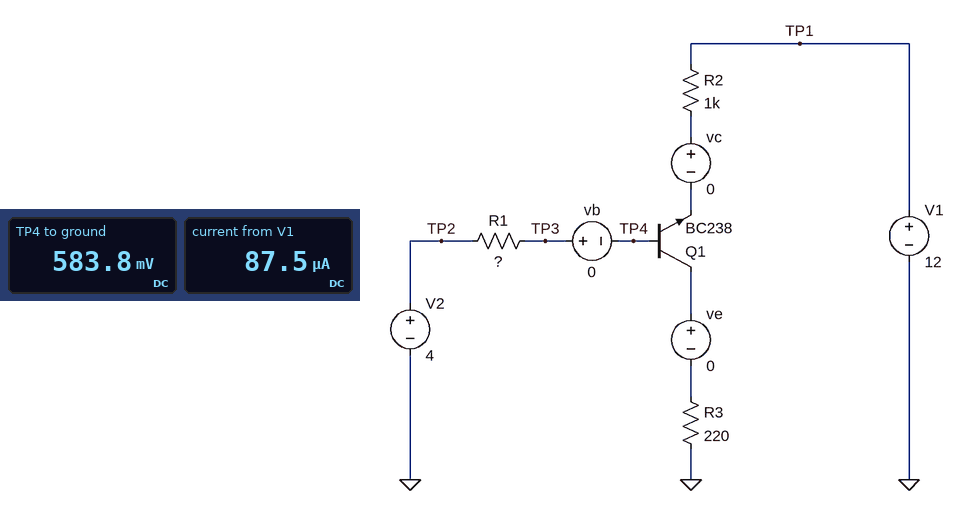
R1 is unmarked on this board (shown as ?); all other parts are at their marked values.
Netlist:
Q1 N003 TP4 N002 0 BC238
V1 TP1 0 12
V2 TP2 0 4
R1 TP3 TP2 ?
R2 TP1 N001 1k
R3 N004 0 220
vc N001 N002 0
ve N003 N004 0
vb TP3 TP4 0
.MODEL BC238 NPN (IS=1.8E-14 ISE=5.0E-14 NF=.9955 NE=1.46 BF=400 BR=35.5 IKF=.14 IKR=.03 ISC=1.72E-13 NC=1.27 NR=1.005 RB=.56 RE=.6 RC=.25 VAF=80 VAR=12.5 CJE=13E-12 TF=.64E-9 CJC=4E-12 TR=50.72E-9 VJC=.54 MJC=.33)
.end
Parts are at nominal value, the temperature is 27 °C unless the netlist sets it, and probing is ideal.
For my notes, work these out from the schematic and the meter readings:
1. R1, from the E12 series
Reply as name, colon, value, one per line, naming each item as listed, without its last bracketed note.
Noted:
R1, from the E12 series: 560 kΩ
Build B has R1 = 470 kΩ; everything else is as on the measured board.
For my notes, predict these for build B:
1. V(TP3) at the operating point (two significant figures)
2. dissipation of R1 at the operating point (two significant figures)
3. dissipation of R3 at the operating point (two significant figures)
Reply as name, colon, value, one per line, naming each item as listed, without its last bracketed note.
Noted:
V(TP3) at the operating point: 590 mV
dissipation of R1 at the operating point: 25 µW
dissipation of R3 at the operating point: 2.9 µW
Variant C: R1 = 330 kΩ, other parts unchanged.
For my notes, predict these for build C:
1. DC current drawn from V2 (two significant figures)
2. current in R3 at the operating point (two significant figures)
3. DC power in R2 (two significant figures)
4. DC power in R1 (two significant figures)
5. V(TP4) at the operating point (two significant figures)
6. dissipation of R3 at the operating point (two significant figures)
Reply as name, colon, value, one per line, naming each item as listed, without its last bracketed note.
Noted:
DC current drawn from V2: 10 µA
current in R3 at the operating point: 170 µA
DC power in R2: 26 µW
DC power in R1: 35 µW
V(TP4) at the operating point: 620 mV
dissipation of R3 at the operating point: 6.5 µW
